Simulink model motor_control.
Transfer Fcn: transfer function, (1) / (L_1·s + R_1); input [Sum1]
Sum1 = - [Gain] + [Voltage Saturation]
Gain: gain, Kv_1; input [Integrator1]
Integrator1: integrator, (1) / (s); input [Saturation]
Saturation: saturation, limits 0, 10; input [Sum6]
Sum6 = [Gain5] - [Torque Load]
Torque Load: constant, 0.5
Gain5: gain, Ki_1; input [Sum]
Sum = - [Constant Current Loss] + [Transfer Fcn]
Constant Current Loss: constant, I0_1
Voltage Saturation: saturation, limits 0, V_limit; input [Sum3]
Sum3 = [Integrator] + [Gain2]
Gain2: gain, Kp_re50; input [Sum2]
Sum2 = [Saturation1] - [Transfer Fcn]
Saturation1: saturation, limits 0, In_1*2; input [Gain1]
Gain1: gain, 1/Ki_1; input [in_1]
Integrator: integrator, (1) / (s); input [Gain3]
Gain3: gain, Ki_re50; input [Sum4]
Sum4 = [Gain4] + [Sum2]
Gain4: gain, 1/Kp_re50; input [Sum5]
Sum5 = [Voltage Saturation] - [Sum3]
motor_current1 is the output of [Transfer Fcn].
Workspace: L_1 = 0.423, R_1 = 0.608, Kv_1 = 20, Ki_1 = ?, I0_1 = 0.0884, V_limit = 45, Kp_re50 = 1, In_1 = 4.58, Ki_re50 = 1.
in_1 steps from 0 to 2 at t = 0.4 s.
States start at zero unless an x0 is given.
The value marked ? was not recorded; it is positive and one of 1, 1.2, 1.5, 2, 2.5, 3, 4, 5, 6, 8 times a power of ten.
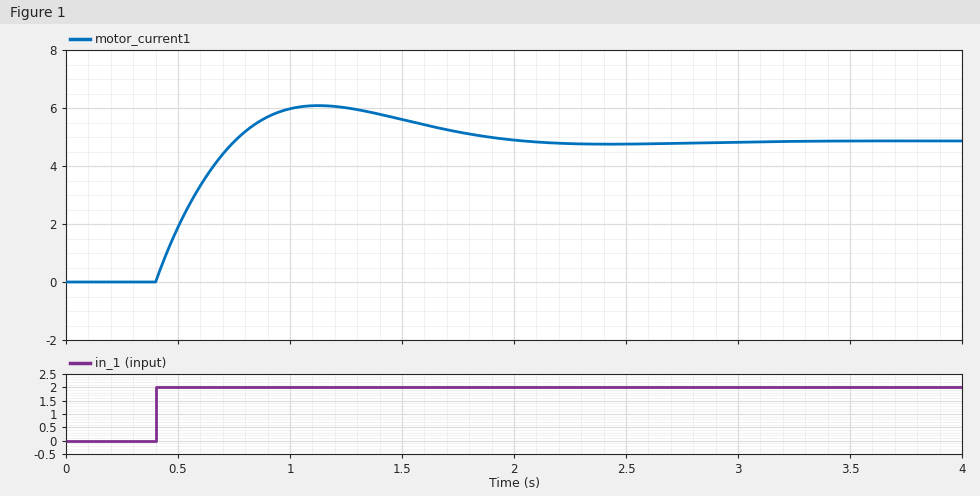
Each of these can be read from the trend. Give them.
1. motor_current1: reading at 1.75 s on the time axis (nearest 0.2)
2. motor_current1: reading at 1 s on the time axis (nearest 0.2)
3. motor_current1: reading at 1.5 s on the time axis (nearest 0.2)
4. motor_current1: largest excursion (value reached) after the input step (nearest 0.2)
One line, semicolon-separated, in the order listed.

5.2; 6.0; 5.6; 6.0
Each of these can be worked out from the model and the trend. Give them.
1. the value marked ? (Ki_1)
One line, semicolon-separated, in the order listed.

0.15
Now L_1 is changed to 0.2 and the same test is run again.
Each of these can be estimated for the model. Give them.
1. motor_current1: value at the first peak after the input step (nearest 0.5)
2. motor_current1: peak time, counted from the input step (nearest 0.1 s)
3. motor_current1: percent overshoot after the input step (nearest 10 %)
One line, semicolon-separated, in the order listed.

6.0; 0.4 s; 120 %
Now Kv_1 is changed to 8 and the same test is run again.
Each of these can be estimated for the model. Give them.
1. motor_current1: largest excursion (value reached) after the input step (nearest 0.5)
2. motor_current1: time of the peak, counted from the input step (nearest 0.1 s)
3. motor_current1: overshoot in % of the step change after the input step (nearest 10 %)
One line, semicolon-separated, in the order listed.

7.0; 1.0 s; 200 %
